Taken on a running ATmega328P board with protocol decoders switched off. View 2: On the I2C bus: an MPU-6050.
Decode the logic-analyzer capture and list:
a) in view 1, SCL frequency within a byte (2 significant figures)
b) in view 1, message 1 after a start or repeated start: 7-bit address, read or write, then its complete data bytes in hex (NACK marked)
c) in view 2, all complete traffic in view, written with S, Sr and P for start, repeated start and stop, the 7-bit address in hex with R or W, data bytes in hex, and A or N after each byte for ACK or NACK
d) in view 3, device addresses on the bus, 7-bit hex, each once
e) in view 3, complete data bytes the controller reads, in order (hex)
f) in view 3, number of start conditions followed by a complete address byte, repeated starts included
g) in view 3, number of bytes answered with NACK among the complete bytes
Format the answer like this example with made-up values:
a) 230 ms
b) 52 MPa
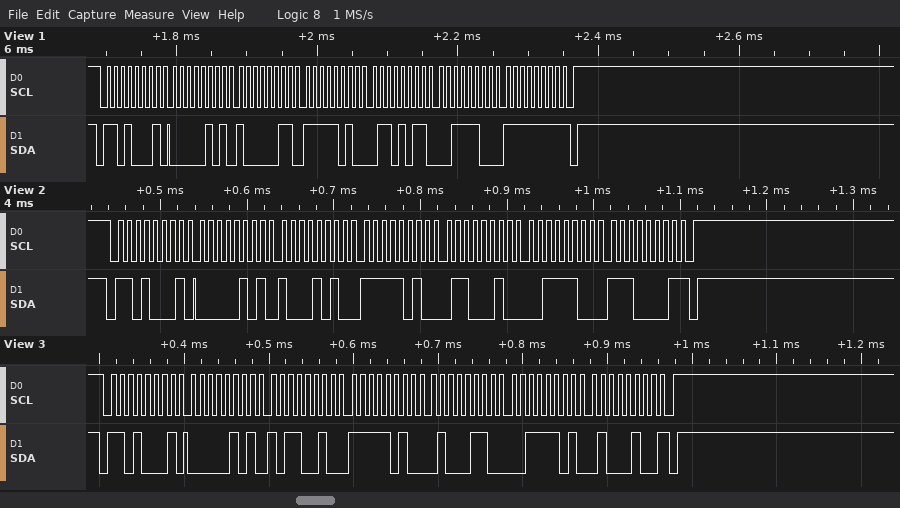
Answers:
a) 100 kHz
b) 0x68 read: 05 83 FA 6B 3C FF NACK
c) S 68R A 05 A 8A A FA A 62 A 3C A E1 N P
d) 0x68
e) 05 B2 FA 46 3D 44
f) 1
g) 1
